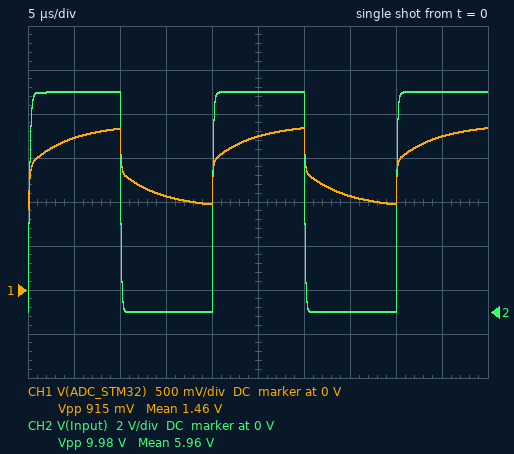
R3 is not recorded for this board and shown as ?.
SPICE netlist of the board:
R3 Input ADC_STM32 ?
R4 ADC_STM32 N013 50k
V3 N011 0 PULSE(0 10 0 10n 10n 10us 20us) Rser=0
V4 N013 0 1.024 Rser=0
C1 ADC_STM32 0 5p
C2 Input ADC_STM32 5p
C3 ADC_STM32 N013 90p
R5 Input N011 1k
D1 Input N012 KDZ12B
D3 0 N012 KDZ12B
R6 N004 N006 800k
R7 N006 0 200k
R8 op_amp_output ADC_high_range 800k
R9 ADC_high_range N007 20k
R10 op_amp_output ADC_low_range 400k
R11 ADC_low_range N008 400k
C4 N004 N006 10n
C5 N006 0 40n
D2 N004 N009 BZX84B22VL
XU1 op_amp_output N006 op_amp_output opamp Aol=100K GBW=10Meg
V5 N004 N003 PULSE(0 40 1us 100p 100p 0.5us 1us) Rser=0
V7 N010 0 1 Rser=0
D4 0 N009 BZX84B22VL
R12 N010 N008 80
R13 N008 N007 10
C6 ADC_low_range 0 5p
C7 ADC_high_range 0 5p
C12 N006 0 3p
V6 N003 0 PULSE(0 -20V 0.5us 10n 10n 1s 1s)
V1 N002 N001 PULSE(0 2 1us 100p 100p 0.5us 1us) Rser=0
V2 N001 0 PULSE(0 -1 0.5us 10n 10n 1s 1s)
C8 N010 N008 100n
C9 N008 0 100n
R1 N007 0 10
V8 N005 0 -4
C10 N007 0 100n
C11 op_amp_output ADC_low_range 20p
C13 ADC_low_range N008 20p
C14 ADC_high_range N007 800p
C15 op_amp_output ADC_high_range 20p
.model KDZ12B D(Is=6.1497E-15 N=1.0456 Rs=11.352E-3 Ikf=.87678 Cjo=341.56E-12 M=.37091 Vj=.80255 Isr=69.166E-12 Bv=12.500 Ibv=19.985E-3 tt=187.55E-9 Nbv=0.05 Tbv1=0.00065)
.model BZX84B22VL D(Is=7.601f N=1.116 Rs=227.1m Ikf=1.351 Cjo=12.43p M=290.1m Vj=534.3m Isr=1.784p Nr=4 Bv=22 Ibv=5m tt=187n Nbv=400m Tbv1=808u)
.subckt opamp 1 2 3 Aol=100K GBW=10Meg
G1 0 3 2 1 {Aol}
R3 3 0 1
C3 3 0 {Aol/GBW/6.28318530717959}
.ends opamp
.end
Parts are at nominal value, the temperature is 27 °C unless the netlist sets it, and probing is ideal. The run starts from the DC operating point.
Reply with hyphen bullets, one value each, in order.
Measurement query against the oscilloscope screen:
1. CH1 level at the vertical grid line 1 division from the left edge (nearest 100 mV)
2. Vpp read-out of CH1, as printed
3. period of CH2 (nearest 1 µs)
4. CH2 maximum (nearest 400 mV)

- 1.7 V
- 915 mV
- 20 µs
- 10.0 V
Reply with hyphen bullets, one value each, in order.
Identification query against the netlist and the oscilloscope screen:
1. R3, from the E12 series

- 470 kΩ
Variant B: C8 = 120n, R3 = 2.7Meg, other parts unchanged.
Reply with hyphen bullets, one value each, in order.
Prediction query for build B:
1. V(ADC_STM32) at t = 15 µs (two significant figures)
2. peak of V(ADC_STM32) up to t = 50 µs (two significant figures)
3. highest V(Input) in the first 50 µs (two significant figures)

- 900 mV
- 1.5 V
- 10 V
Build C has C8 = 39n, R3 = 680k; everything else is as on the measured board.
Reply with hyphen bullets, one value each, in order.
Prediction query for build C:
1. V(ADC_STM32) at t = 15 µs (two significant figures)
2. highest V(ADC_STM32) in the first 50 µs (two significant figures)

- 1.0 V
- 1.6 V
